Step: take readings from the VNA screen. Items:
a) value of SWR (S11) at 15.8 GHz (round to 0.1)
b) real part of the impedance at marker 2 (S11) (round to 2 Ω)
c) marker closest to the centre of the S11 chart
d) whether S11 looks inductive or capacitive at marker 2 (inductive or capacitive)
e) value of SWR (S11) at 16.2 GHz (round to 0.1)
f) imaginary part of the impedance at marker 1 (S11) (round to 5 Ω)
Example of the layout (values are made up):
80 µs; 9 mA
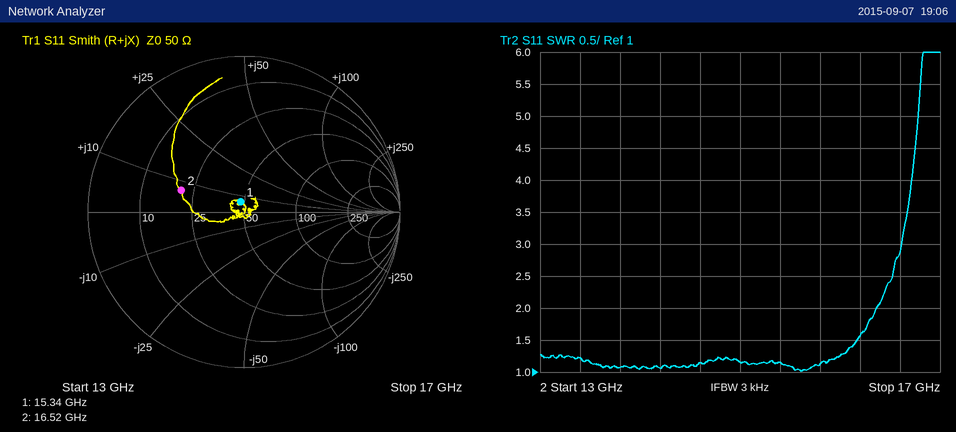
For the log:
1.1; 20 Ω; marker 1; inductive; 1.6; +5 Ω
